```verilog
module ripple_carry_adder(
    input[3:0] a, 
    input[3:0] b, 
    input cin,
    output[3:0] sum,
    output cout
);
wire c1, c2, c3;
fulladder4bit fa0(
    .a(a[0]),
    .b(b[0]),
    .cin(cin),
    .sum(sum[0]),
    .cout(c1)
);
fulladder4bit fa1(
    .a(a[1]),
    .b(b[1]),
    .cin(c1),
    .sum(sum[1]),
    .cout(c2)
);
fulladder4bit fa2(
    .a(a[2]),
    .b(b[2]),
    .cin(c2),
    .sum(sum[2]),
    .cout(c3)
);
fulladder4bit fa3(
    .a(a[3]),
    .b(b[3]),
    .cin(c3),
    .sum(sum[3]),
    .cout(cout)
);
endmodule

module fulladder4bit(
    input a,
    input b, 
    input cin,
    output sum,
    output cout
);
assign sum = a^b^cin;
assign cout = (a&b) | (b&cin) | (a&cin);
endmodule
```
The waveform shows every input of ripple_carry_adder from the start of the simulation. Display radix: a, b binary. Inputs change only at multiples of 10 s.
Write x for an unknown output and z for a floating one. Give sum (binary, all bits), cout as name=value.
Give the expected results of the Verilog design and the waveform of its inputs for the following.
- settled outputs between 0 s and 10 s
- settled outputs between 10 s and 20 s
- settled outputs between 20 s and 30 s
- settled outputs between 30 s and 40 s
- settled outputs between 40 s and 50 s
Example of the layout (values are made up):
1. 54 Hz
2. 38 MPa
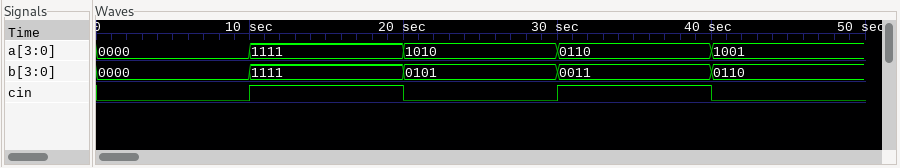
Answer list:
1. sum=0000, cout=0
2. sum=1111, cout=1
3. sum=1111, cout=0
4. sum=1010, cout=0
5. sum=1111, cout=0
